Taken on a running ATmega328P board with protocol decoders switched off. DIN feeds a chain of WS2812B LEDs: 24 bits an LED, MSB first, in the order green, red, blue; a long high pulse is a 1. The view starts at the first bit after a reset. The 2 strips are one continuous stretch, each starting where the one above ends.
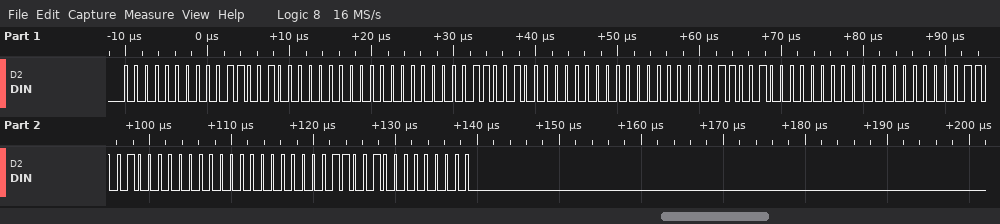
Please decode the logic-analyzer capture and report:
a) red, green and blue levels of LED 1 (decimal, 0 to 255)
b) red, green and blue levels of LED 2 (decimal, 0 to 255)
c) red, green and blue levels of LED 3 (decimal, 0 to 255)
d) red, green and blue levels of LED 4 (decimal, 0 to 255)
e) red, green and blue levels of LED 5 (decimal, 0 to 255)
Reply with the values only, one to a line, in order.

50, 0, 0
50, 0, 0
50, 0, 0
50, 0, 0
50, 0, 0
